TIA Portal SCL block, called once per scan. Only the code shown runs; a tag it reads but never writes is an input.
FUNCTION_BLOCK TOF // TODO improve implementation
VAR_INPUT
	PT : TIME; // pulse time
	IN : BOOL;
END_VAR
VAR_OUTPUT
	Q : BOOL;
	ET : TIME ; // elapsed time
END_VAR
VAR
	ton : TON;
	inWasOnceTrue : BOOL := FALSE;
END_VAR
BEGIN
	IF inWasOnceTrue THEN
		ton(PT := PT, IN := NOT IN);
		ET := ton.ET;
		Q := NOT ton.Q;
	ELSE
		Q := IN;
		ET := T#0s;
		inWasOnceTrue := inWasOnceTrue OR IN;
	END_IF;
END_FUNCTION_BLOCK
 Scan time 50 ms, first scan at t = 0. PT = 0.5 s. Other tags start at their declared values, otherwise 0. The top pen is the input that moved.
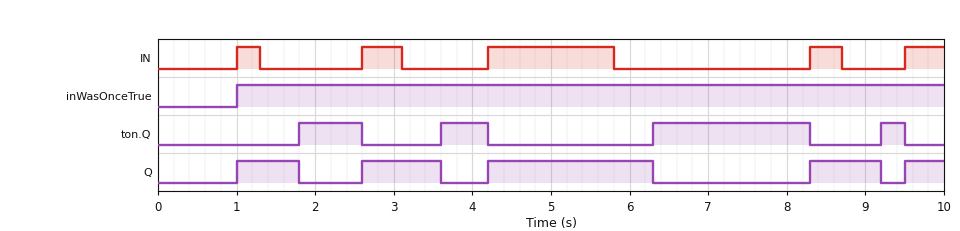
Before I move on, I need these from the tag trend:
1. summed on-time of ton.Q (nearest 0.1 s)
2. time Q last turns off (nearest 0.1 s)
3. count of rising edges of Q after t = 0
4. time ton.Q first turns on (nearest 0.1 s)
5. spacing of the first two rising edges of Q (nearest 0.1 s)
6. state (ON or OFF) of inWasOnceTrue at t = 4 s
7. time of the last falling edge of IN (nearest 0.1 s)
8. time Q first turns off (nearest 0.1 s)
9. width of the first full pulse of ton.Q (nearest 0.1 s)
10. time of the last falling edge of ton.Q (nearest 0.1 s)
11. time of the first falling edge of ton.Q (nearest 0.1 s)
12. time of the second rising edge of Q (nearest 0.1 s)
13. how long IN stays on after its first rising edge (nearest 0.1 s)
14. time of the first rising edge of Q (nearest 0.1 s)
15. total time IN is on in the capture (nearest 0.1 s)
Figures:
3.7 s
9.2 s
5
1.8 s
1.6 s
ON
8.7 s
1.8 s
0.8 s
9.5 s
2.6 s
2.6 s
0.3 s
1.0 s
3.3 s
